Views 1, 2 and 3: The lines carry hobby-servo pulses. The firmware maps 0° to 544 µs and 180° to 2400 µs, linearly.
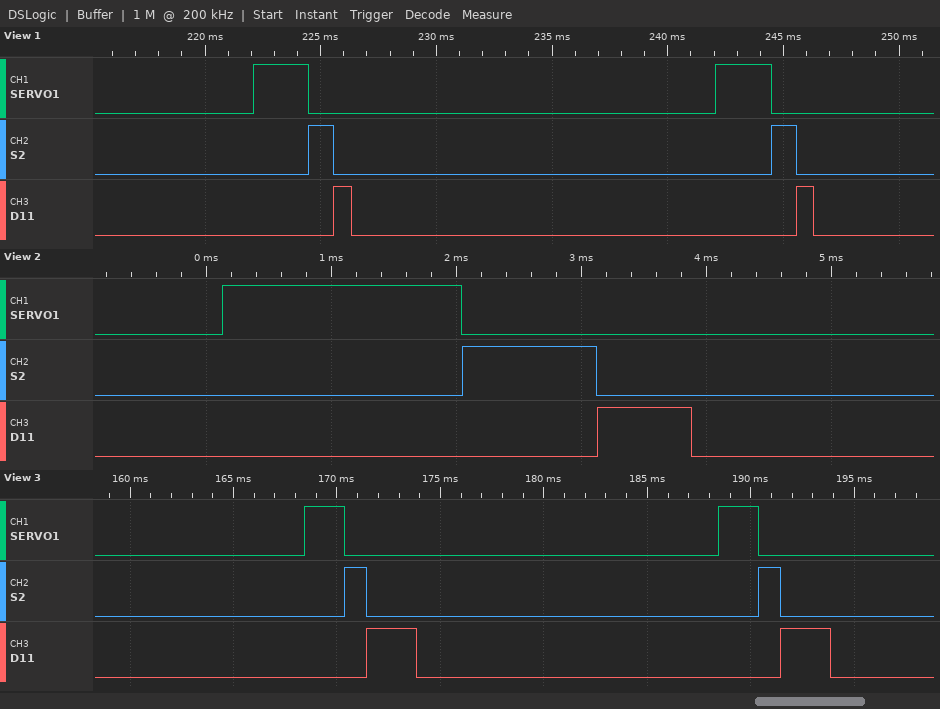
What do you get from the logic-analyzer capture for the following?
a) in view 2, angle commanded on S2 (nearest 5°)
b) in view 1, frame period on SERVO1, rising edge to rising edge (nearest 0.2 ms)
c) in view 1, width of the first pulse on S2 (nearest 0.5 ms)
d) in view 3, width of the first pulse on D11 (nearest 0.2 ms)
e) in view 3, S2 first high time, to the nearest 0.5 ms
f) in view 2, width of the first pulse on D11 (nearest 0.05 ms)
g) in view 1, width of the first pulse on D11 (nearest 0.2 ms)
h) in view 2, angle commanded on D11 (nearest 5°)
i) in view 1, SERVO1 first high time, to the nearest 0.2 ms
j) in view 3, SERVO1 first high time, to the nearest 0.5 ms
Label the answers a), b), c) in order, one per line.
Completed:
a) 50°
b) 20.0 ms
c) 1.0 ms
d) 2.4 ms
e) 1.0 ms
f) 0.75 ms
g) 0.8 ms
h) 20°
i) 2.4 ms
j) 2.0 ms
